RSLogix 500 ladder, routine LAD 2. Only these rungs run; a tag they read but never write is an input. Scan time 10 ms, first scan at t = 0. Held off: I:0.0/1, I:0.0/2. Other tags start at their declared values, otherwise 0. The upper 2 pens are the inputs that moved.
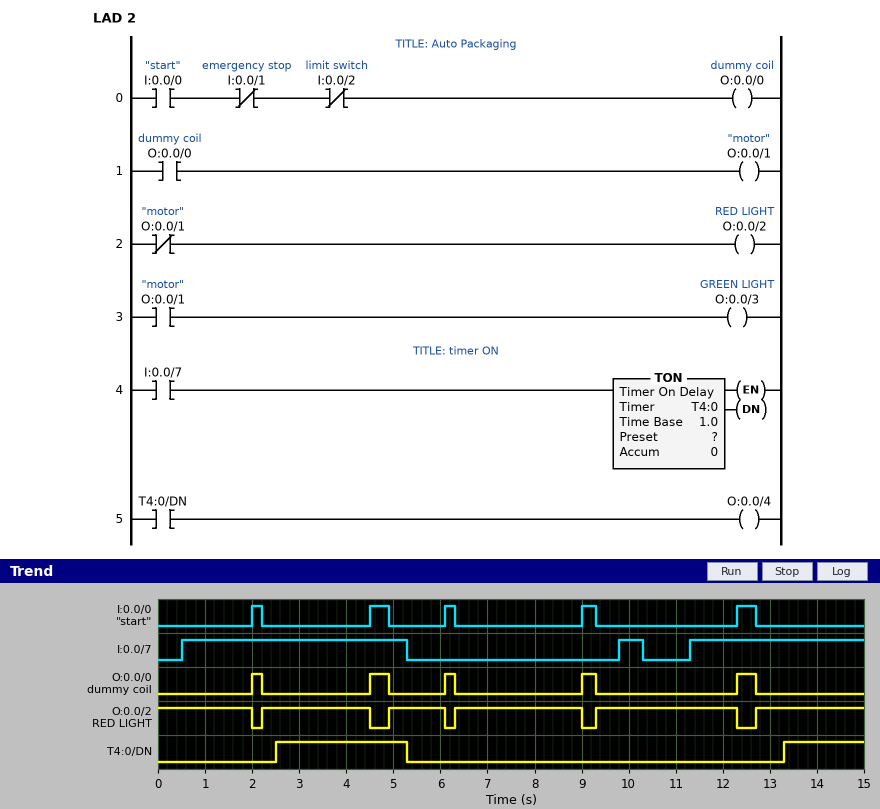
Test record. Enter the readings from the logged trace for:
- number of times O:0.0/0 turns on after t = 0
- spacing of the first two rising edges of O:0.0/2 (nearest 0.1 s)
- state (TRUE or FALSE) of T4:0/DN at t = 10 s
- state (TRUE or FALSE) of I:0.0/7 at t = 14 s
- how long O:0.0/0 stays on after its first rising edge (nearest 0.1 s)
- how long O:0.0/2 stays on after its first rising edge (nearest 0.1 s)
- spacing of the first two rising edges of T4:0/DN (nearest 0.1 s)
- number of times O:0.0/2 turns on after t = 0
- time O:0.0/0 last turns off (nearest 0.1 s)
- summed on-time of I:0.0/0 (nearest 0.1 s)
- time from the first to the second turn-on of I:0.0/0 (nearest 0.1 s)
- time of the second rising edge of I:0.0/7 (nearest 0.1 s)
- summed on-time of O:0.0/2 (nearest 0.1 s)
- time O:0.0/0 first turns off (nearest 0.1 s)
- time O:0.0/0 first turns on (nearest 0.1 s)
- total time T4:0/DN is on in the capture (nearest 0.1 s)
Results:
5
2.7 s
FALSE
TRUE
0.2 s
2.3 s
10.8 s
5
12.7 s
1.5 s
2.5 s
9.8 s
13.5 s
2.2 s
2.0 s
4.5 s
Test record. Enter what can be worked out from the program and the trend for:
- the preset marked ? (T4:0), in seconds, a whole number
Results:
2 s
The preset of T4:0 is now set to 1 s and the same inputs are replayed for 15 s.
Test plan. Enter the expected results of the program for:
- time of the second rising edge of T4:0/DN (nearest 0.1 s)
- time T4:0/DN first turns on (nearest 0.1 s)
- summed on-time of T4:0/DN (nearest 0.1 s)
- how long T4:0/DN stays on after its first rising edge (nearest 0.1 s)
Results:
12.3 s
1.5 s
6.5 s
3.8 s
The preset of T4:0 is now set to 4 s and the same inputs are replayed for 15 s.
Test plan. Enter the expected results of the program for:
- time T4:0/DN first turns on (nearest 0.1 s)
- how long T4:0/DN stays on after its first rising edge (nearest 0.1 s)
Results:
4.5 s
0.8 s
